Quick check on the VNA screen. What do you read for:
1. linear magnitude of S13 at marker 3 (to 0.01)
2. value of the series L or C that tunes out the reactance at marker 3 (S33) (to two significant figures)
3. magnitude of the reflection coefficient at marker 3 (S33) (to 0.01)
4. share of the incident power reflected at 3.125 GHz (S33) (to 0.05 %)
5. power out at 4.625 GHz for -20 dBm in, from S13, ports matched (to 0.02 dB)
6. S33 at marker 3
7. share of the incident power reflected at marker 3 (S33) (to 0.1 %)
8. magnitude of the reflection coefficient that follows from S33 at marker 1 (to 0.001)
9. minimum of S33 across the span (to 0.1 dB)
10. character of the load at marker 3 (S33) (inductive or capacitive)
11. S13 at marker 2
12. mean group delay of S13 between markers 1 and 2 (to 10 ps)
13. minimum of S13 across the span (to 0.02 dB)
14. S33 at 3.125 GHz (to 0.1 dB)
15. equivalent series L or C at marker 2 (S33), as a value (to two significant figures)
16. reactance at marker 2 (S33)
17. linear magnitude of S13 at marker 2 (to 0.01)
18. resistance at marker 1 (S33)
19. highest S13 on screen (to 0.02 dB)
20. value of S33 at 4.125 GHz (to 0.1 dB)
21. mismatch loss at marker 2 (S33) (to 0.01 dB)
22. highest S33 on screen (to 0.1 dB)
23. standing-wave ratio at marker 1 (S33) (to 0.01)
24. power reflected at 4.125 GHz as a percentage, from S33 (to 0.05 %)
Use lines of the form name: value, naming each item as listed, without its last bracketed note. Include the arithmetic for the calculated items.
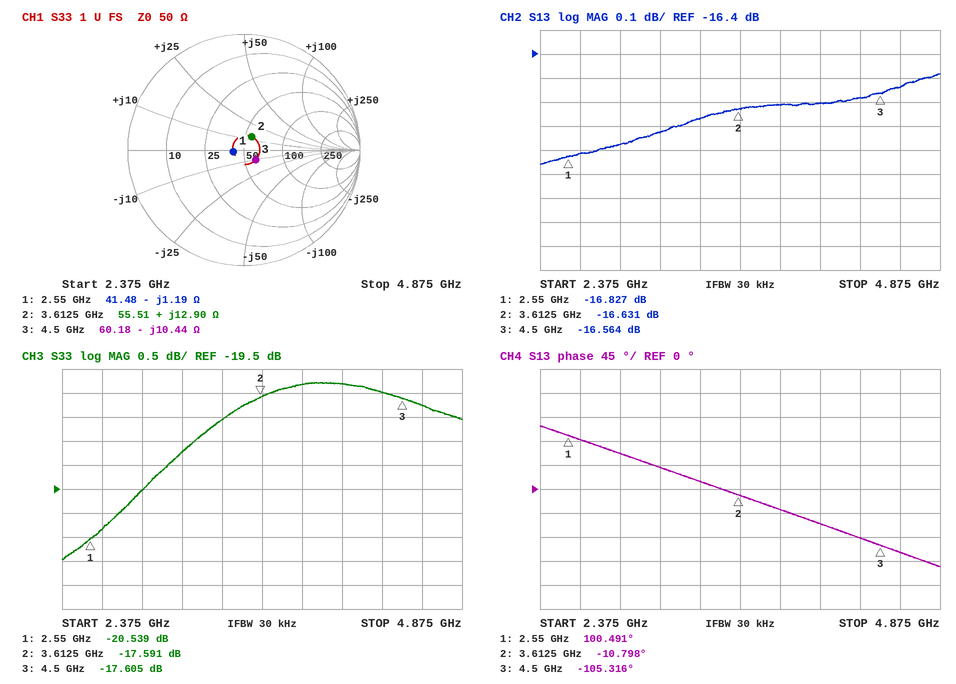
linear magnitude of S13 at marker 3: 10^(-16.564/20) ≈ 0.15
value of the series L or C that tunes out the reactance at marker 3 (S33): L = 10.44 Ω/(2π × 4.5 GHz) ≈ 369 pH, so 370 pH to two significant figures
magnitude of the reflection coefficient at marker 3 (S33): 0.13
share of the incident power reflected at 3.125 GHz (S33): 10^(-18.7/10) ≈ 1.35 %
power out at 4.625 GHz for -20 dBm in, from S13, ports matched: -20 dBm + (-16.54 dB) = -36.54 dBm
S33 at marker 3: -17.605 dB
share of the incident power reflected at marker 3 (S33): 10^(-17.605/10) ≈ 1.7 %
magnitude of the reflection coefficient that follows from S33 at marker 1: 10^(-20.539/20) ≈ 0.094
minimum of S33 across the span: -21.0 dB
character of the load at marker 3 (S33): capacitive
S13 at marker 2: -16.631 dB
mean group delay of S13 between markers 1 and 2: −(-10.798° − (100.491°))/(360° × 1.0625 GHz) ≈ 291 ps, so 290 ps to the nearest 10 ps
minimum of S13 across the span: -16.86 dB
S33 at 3.125 GHz: -18.7 dB
equivalent series L or C at marker 2 (S33), as a value: L = 12.9 Ω/(2π × 3.6125 GHz) ≈ 568 pH, so 570 pH to two significant figures
reactance at marker 2: +12.90 Ω
linear magnitude of S13 at marker 2: 10^(-16.631/20) ≈ 0.15
resistance at marker 1: 41.48 Ω
highest S13 on screen: -16.48 dB
value of S33 at 4.125 GHz: -17.3 dB
mismatch loss at marker 2 (S33): −10 log10(1 − 10^(-17.591/10)) ≈ 0.08 dB
highest S33 on screen: -17.3 dB
standing-wave ratio at marker 1 (S33): 1.21
power reflected at 4.125 GHz as a percentage, from S33: 10^(-17.3/10) ≈ 1.86 %, so 1.85 % to the nearest 0.05 %
